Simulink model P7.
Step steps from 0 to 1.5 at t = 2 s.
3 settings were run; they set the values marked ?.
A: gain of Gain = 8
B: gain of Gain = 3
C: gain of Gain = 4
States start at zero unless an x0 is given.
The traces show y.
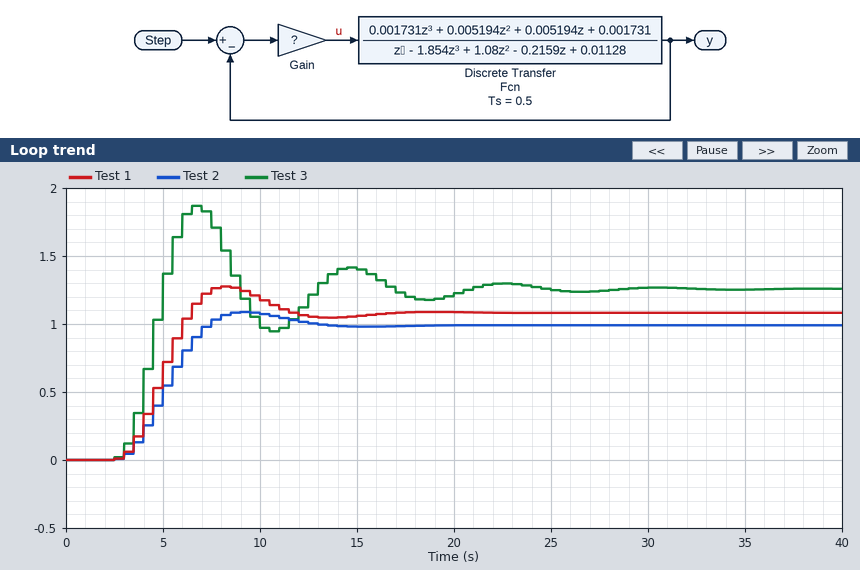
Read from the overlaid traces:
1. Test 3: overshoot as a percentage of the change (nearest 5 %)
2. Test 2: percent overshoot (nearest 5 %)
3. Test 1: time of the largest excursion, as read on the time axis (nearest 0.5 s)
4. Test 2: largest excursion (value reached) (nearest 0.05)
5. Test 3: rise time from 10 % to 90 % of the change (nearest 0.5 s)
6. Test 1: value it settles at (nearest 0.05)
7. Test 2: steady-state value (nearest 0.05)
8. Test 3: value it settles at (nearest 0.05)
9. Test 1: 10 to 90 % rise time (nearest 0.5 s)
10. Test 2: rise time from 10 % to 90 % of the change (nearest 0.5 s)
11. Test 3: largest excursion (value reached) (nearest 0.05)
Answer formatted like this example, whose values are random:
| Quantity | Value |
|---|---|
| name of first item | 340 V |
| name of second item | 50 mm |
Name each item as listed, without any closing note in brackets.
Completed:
| Quantity | Value |
|---|---|
| Test 3: overshoot as a percentage of the change | 50 % |
| Test 2: percent overshoot | 10 % |
| Test 1: time of the largest excursion, as read on the time axis | 8.0 s |
| Test 2: largest excursion (value reached) | 1.10 |
| Test 3: rise time from 10 % to 90 % of the change | 1.5 s |
| Test 1: value it settles at | 1.10 |
| Test 2: steady-state value | 1.00 |
| Test 3: value it settles at | 1.25 |
| Test 1: 10 to 90 % rise time | 2.5 s |
| Test 2: rise time from 10 % to 90 % of the change | 3.0 s |
| Test 3: largest excursion (value reached) | 1.85 |
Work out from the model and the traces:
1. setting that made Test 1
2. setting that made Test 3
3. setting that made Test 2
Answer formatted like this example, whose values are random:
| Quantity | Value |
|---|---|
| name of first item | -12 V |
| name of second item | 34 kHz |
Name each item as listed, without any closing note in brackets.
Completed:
| Quantity | Value |
|---|---|
| setting that made Test 1 | C |
| setting that made Test 3 | A |
| setting that made Test 2 | B |
